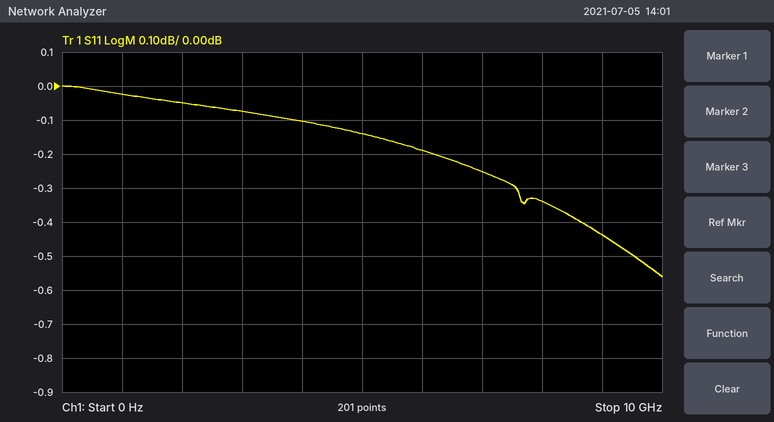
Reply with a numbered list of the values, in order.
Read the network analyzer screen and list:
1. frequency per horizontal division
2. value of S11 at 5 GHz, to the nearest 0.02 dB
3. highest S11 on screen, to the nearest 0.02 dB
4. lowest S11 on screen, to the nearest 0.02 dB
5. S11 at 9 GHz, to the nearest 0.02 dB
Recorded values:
1. 1 GHz
2. -0.14 dB
3. 0.00 dB
4. -0.56 dB
5. -0.44 dB
